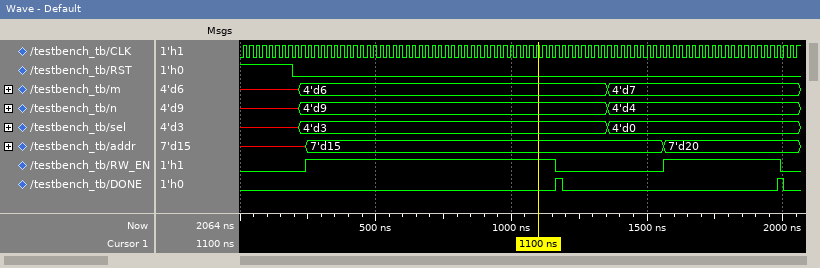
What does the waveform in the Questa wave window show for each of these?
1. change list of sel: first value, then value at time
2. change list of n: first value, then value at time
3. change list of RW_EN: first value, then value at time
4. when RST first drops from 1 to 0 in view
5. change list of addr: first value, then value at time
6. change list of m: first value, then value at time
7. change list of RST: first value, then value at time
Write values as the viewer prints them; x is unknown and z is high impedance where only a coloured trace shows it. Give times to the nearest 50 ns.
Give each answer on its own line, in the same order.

x, 4'd3 at 200 ns, 4'd0 at 1350 ns
x, 4'd9 at 200 ns, 4'd4 at 1350 ns
0, 1 at 250 ns, 0 at 1150 ns, 1 at 1550 ns, 0 at 2000 ns
200 ns
x, 7'd15 at 250 ns, 7'd20 at 1550 ns
x, 4'd6 at 200 ns, 4'd7 at 1350 ns
1, 0 at 200 ns
